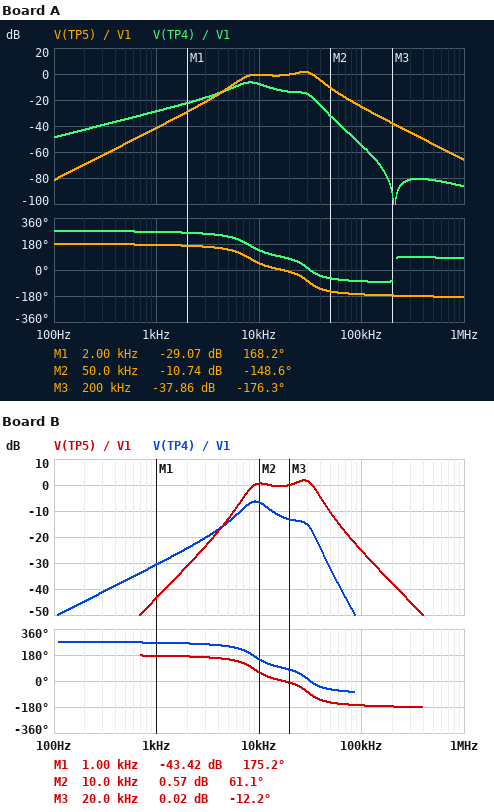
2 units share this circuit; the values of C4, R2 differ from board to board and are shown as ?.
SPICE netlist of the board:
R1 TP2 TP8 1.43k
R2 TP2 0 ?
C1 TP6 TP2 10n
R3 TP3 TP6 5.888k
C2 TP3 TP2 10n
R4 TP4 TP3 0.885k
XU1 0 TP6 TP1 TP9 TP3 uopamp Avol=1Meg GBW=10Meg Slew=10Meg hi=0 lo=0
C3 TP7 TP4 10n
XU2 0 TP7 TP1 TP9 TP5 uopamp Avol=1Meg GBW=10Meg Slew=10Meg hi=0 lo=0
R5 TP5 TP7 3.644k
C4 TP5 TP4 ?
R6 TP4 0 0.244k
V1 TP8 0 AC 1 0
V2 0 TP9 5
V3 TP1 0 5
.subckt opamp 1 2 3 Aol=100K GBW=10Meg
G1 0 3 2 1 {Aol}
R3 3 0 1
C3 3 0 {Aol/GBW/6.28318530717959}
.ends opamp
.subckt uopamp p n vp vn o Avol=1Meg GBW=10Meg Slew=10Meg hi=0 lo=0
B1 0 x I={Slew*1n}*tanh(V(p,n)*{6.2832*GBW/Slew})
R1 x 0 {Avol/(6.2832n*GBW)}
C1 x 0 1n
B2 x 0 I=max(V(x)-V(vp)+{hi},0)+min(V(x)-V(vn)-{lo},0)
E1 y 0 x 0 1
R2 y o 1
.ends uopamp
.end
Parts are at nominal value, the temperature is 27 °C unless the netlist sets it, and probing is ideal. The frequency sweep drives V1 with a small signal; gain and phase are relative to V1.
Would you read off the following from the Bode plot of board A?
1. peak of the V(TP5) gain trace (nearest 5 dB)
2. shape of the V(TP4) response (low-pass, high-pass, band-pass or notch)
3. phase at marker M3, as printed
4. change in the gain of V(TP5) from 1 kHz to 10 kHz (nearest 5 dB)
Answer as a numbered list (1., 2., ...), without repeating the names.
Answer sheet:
1. 0 dB
2. band-pass
3. -176.3 deg
4. 40 dB
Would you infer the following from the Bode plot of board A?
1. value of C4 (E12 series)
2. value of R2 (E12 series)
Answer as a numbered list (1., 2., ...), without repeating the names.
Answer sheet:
1. 3.9 nF
2. 1.2 kΩ
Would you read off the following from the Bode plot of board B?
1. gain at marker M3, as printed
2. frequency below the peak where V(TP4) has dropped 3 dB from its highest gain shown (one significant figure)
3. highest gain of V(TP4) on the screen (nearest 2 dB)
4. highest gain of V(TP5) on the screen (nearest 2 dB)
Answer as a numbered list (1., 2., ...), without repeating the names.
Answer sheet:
1. 0.02 dB
2. 7 kHz
3. -6 dB
4. 2 dB
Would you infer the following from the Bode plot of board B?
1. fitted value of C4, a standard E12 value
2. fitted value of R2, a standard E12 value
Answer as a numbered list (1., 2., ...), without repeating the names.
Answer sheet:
1. 3.9 nF
2. 820 Ω
